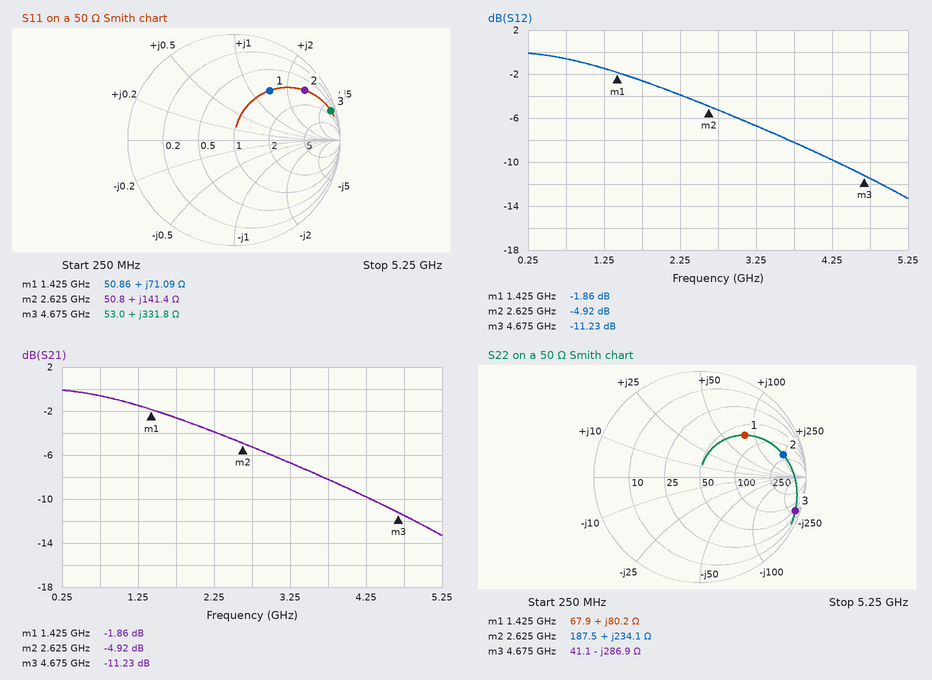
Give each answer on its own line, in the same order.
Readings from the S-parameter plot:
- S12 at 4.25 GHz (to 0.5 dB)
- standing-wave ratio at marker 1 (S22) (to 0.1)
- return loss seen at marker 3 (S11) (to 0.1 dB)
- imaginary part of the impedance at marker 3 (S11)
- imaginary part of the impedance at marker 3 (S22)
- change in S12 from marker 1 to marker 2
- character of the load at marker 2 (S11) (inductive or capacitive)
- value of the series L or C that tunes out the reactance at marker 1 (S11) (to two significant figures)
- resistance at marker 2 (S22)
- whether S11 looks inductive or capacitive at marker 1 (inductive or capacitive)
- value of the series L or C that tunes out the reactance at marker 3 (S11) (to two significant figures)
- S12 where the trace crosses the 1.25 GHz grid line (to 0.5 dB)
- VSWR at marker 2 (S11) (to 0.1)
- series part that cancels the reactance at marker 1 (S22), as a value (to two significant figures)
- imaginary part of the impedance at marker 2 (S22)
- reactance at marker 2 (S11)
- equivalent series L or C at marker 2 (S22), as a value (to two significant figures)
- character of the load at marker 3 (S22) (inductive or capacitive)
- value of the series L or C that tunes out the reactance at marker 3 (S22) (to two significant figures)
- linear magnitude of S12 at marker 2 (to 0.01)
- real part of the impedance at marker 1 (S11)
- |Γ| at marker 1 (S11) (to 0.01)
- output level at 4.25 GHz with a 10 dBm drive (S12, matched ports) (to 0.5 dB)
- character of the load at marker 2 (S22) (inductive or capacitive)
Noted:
-10.0 dB
3.7
0.4 dB
+331.8 Ω
-286.9 Ω
-3.06 dB
inductive
1.6 pF
187.5 Ω
inductive
100 fF
-1.5 dB
9.8
1.4 pF
+234.1 Ω
+141.4 Ω
14 nH
capacitive
9.8 nH
0.57
50.86 Ω
0.58
0.0 dBm
inductive
